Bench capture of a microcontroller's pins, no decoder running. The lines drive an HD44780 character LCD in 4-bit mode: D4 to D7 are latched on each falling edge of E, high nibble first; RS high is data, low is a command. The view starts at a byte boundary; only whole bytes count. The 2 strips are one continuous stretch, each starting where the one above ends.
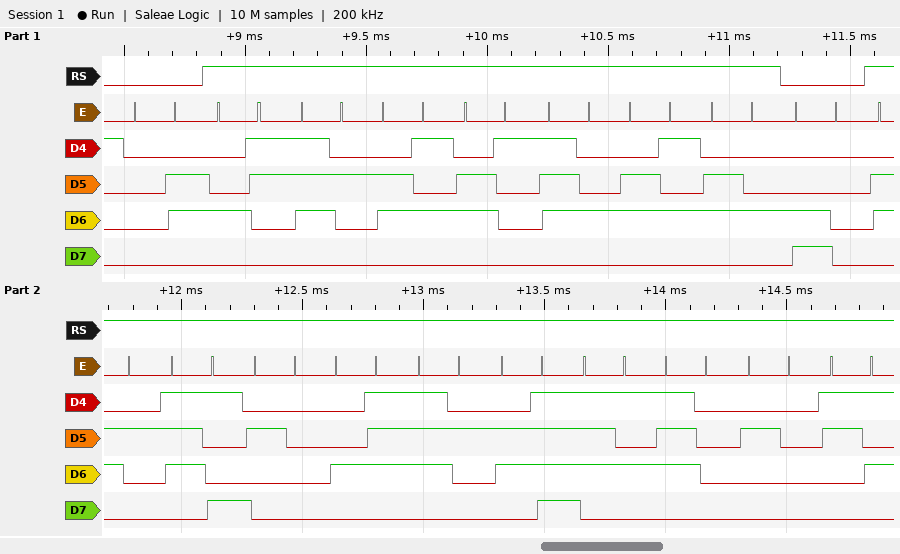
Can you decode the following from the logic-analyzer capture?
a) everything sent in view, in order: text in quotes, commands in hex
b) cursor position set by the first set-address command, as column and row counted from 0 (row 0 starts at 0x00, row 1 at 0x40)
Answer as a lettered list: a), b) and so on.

a) 0x06 "Created" 0xC0 "by Group 5"
b) column 0, row 1
